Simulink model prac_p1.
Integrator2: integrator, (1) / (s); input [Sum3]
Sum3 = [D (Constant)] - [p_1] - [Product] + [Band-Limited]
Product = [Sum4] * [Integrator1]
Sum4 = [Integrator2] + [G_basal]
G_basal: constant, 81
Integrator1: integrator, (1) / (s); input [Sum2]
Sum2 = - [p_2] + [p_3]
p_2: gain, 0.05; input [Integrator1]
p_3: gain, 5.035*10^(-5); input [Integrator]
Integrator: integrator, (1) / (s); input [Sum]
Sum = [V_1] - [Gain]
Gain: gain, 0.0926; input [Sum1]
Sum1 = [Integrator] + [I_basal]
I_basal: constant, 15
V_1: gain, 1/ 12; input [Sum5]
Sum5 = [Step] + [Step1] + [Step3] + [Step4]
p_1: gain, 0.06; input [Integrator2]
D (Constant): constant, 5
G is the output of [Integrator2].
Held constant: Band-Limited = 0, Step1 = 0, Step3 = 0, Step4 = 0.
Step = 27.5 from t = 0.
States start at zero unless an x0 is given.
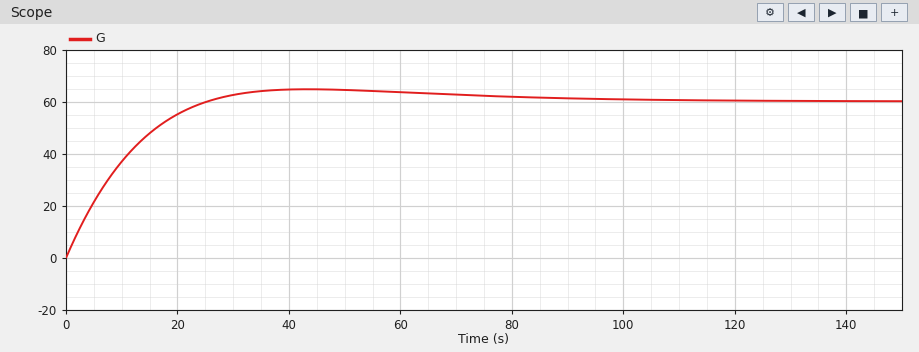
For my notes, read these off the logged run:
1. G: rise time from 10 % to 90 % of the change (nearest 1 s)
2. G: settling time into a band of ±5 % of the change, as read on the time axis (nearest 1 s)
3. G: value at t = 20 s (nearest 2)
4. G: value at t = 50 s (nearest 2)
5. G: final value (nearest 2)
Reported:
18 s
65 s
56
64
60
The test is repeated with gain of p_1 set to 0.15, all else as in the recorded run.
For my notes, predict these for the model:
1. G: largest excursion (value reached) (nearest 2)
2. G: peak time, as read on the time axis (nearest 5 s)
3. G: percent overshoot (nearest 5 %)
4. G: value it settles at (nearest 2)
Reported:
30
25 s
15 %
26
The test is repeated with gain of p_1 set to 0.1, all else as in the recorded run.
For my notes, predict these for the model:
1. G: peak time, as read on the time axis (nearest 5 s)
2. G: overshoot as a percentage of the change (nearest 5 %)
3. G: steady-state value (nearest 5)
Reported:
30 s
10 %
40
